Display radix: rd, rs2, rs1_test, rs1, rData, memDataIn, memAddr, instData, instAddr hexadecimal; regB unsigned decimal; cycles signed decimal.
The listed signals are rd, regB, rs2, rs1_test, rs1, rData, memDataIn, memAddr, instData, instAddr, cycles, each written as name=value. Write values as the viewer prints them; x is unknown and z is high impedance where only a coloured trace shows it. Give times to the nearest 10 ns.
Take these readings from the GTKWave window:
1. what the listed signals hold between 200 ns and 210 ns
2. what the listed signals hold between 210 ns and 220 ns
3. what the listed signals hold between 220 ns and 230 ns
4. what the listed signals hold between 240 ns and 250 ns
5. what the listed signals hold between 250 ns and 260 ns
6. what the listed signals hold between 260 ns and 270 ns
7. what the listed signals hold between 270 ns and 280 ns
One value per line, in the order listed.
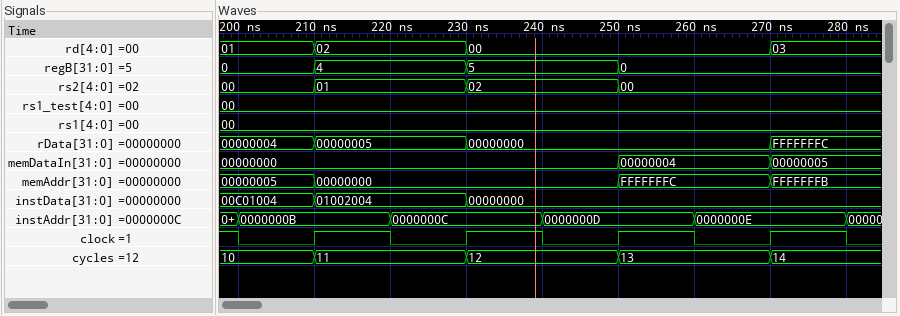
rd=01, regB=0, rs2=00, rs1_test=00, rs1=00, rData=00000004, memDataIn=00000000, memAddr=00000005, instData=00C01004, instAddr=0000000B, cycles=10
rd=02, regB=4, rs2=01, rs1_test=00, rs1=00, rData=00000005, memDataIn=00000000, memAddr=00000000, instData=01002004, instAddr=0000000B, cycles=11
rd=02, regB=4, rs2=01, rs1_test=00, rs1=00, rData=00000005, memDataIn=00000000, memAddr=00000000, instData=01002004, instAddr=0000000C, cycles=11
rd=00, regB=5, rs2=02, rs1_test=00, rs1=00, rData=00000000, memDataIn=00000000, memAddr=00000000, instData=00000000, instAddr=0000000D, cycles=12
rd=00, regB=0, rs2=00, rs1_test=00, rs1=00, rData=00000000, memDataIn=00000004, memAddr=FFFFFFFC, instData=00000000, instAddr=0000000D, cycles=13
rd=00, regB=0, rs2=00, rs1_test=00, rs1=00, rData=00000000, memDataIn=00000004, memAddr=FFFFFFFC, instData=00000000, instAddr=0000000E, cycles=13
rd=03, regB=0, rs2=00, rs1_test=00, rs1=00, rData=FFFFFFFC, memDataIn=00000005, memAddr=FFFFFFFB, instData=00000000, instAddr=0000000E, cycles=14
